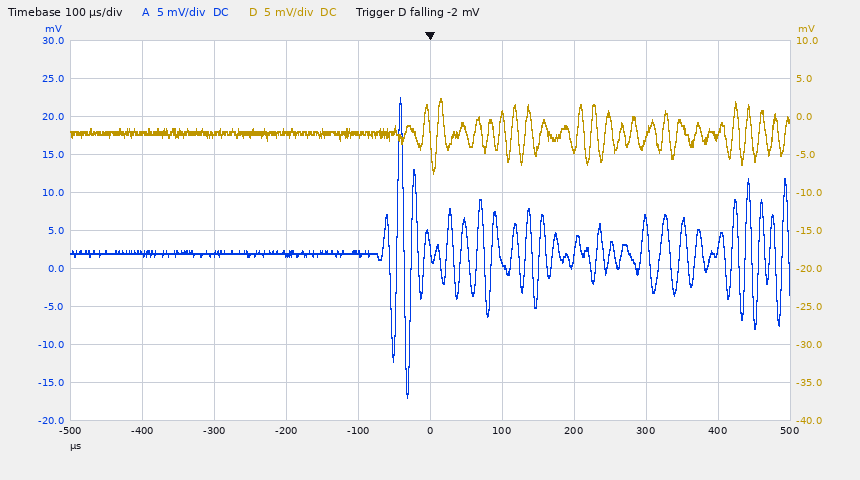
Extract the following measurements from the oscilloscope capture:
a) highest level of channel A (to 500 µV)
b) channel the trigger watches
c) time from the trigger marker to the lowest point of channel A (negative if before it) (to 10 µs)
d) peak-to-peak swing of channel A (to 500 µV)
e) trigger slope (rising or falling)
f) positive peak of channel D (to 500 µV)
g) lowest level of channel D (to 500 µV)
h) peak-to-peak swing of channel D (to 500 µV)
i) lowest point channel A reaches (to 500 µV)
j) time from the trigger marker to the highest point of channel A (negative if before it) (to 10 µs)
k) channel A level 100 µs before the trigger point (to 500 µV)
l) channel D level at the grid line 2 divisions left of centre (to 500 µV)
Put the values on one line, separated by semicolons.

22.5 mV; channel D; -30 µs; 39.5 mV; falling; 2.5 mV; -7.5 mV; 10.0 mV; -17.0 mV; -40 µs; 2.0 mV; -2.0 mV
